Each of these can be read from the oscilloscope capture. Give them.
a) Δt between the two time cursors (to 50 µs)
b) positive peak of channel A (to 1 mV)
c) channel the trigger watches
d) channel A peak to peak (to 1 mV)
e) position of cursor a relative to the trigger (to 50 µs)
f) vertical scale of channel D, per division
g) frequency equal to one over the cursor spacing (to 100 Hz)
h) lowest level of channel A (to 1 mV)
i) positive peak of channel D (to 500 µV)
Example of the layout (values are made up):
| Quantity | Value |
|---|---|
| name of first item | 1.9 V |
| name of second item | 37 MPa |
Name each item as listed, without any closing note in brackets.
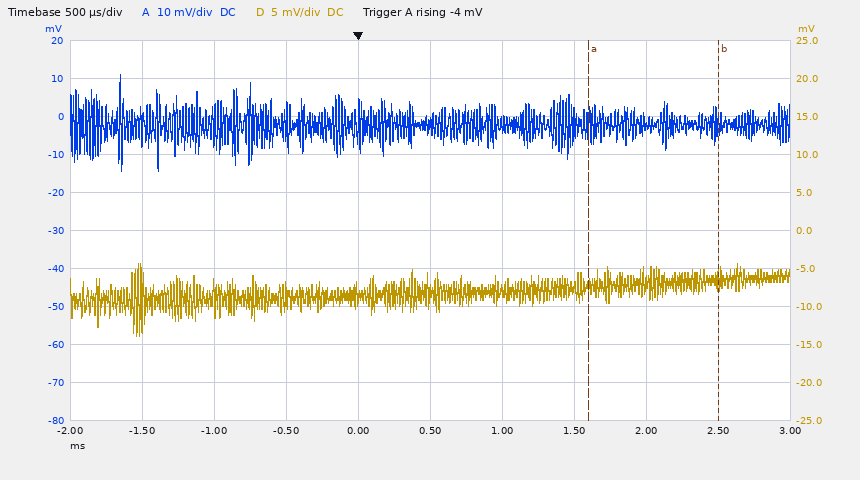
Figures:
| Quantity | Value |
|---|---|
| Δt between the two time cursors | 900 µs |
| positive peak of channel A | 11 mV |
| channel the trigger watches | channel A |
| channel A peak to peak | 25 mV |
| position of cursor a relative to the trigger | +1.60 ms |
| vertical scale of channel D, per division | 5 mV |
| frequency equal to one over the cursor spacing | 1.1 kHz |
| lowest level of channel A | -14 mV |
| positive peak of channel D | -4.5 mV |
